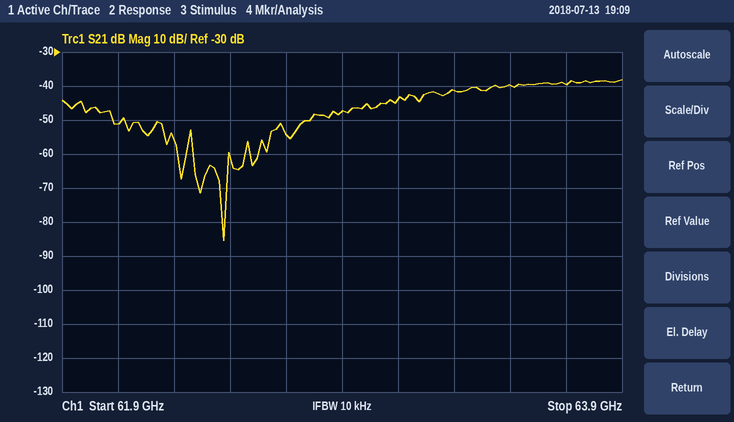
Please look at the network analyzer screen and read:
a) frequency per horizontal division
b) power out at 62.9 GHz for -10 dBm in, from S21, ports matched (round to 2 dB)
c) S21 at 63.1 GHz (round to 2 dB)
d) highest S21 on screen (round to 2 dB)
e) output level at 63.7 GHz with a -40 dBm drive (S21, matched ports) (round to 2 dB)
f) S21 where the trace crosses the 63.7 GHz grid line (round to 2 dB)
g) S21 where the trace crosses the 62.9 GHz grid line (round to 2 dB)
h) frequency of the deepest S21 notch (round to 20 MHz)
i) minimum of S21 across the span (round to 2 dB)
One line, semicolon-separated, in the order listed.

200 MHz; -58 dBm; -44 dB; -38 dB; -80 dBm; -40 dB; -48 dB; 62.48 GHz; -86 dB
